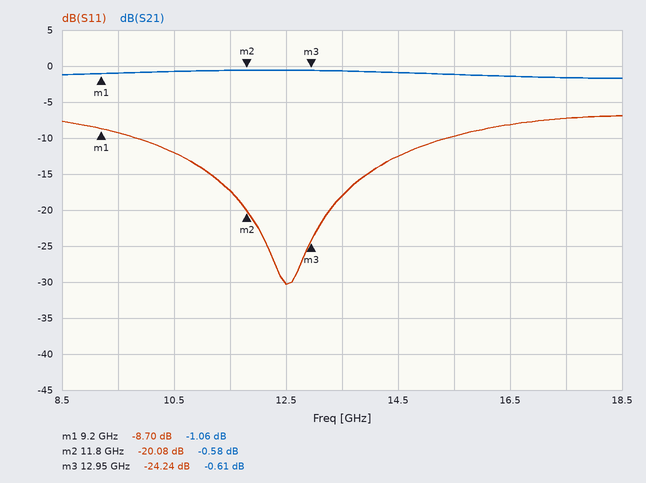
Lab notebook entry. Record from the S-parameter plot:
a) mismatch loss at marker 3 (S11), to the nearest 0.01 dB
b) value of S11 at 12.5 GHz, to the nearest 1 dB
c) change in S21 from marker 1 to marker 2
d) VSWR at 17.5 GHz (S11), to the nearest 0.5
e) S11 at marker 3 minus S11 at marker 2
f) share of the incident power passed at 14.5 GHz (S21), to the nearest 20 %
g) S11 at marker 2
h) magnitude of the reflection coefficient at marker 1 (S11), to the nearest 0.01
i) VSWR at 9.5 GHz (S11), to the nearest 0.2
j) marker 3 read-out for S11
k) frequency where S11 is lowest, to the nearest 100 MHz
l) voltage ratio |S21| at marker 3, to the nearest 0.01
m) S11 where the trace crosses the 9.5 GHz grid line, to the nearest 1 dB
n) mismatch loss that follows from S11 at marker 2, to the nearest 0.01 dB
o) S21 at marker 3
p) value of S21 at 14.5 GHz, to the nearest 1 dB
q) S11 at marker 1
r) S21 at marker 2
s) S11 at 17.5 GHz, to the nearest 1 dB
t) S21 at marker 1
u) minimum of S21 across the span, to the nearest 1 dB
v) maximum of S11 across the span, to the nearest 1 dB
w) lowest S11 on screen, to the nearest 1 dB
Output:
0.02 dB
-30 dB
0.48 dB
2.5
-4.16 dB
80 %
-20.08 dB
0.37
2.0
-24.24 dB
12.5 GHz
0.93
-9 dB
0.04 dB
-0.61 dB
-1 dB
-8.70 dB
-0.58 dB
-7 dB
-1.06 dB
-2 dB
-7 dB
-30 dB
